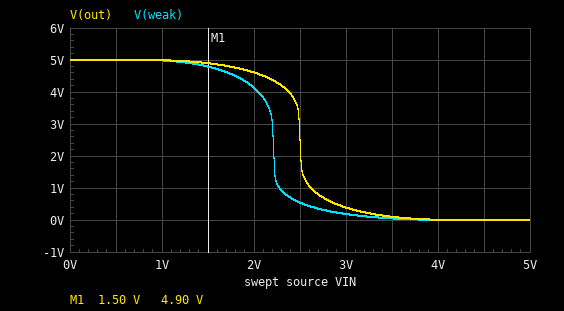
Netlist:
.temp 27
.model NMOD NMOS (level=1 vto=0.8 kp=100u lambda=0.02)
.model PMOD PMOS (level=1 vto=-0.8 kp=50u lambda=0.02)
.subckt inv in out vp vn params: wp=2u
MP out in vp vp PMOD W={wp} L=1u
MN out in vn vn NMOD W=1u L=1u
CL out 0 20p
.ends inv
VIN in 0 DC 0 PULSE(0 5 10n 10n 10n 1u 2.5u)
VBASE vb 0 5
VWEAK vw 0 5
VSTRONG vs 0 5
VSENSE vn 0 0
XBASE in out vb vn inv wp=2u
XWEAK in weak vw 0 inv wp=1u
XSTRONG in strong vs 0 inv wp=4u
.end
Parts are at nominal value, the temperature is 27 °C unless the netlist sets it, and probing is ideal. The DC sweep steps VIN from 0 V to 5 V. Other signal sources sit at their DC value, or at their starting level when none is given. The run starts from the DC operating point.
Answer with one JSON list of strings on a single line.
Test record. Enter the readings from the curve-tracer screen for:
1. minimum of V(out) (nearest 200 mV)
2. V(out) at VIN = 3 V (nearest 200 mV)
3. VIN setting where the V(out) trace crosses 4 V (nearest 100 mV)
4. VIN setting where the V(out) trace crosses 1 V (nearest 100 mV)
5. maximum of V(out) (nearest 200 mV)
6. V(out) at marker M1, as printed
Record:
["0 V", "400 mV", "2.4 V", "2.6 V", "5.0 V", "4.90 V"]
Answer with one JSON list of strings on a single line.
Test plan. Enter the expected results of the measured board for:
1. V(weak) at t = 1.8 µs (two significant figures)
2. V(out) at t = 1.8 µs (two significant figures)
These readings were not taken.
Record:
["5.0 V", "5.0 V"]
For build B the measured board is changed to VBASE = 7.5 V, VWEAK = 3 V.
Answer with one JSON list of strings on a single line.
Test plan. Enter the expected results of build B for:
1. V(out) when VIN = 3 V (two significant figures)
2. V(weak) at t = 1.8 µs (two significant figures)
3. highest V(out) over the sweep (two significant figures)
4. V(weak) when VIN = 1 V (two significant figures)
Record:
["6.7 V", "2.9 V", "7.5 V", "3.0 V"]
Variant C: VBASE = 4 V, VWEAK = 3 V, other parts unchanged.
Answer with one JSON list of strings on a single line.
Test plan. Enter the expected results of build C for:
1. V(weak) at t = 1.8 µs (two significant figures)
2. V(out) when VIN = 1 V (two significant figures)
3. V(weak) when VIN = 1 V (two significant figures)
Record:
["2.9 V", "4.0 V", "3.0 V"]
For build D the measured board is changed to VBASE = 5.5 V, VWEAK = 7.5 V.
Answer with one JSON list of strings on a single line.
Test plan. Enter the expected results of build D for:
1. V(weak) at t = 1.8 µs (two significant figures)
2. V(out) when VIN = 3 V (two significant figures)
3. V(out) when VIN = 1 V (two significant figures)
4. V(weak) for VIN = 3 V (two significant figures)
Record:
["7.5 V", "880 mV", "5.5 V", "5.6 V"]
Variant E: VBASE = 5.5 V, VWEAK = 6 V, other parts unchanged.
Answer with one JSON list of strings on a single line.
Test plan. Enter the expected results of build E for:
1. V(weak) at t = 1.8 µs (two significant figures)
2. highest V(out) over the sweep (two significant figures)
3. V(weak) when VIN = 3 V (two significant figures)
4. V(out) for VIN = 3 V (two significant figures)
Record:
["6.0 V", "5.5 V", "720 mV", "880 mV"]
